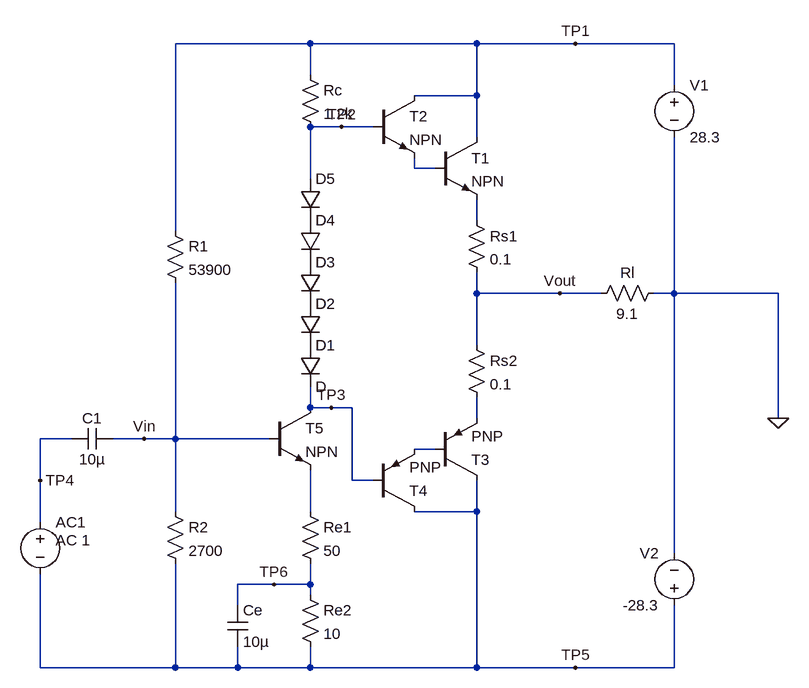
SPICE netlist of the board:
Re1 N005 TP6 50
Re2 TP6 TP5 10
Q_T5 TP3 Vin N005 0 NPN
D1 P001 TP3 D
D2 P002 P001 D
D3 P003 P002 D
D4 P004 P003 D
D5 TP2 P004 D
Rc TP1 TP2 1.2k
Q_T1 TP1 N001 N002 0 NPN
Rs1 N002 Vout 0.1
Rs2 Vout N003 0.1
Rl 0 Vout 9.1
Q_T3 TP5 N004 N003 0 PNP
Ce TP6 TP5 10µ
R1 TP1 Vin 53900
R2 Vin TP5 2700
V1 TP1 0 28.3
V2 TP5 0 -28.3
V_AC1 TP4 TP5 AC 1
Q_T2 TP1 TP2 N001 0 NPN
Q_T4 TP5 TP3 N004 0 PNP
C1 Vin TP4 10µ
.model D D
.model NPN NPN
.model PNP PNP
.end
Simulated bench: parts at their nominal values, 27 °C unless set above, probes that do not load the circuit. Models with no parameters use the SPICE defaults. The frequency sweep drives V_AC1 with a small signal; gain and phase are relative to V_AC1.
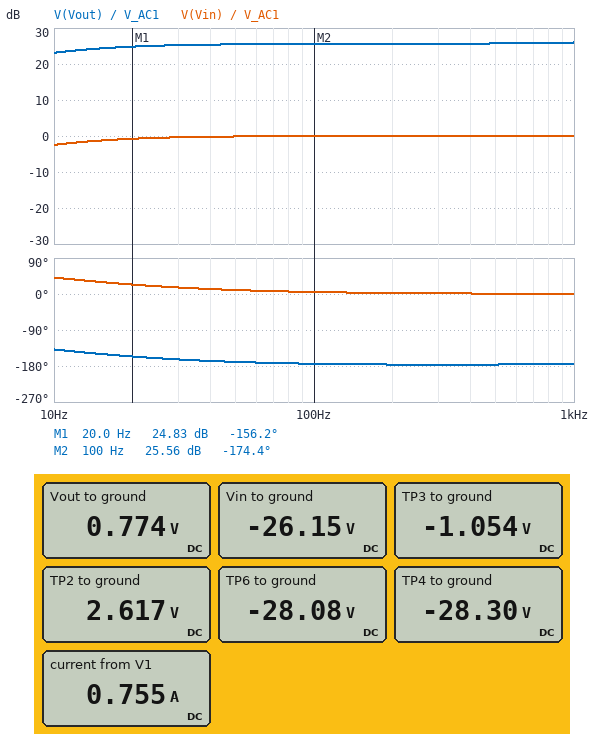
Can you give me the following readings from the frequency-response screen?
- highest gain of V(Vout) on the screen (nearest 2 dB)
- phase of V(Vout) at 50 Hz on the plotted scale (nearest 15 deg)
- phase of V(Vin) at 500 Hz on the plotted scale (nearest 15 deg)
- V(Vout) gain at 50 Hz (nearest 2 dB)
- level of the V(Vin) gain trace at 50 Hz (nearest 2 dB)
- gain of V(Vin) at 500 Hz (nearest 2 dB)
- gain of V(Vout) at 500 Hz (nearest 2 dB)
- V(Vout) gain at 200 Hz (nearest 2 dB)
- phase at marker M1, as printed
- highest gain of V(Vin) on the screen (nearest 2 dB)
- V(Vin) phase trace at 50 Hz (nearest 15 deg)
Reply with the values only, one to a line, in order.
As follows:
26 dB
-165 deg
0 deg
26 dB
0 dB
0 dB
26 dB
26 dB
-156.2 deg
0 dB
15 deg
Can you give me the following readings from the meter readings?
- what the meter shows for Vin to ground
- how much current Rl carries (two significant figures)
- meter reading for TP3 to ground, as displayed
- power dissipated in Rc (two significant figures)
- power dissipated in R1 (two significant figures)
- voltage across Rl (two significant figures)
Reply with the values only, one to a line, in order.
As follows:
-26.15 V
85 mA
-1.054 V
550 mW
55 mW
770 mV
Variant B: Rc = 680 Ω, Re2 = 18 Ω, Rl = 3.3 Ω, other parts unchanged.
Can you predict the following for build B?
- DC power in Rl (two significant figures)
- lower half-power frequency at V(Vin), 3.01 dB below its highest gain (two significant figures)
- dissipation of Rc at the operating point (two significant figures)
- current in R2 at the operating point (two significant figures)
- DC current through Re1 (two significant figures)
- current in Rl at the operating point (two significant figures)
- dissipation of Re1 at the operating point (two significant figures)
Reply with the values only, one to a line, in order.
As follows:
47 W
8.5 Hz
270 mW
810 µA
20 mA
3.8 A
20 mW
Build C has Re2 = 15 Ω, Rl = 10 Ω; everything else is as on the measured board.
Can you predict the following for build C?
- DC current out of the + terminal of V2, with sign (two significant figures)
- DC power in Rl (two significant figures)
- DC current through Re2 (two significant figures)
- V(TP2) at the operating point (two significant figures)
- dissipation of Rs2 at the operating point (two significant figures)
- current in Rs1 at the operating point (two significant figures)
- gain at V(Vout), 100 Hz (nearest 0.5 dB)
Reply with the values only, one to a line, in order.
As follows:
-590 mA
460 mW
20 mA
4.0 V
32 mW
780 mA
25.0 dB
